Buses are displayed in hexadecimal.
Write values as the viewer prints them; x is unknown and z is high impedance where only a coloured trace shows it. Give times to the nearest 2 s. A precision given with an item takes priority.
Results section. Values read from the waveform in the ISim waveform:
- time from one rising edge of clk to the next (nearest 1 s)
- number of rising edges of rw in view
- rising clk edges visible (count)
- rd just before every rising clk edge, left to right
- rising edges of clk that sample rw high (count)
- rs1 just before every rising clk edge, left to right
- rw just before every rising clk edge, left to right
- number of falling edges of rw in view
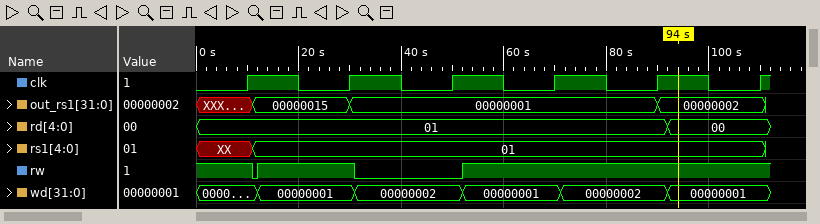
20 s
2
6
01, 01, 01, 01, 01, 00
5
XX, 01, 01, 01, 01, 01
1 1 0 1 1 1
2
